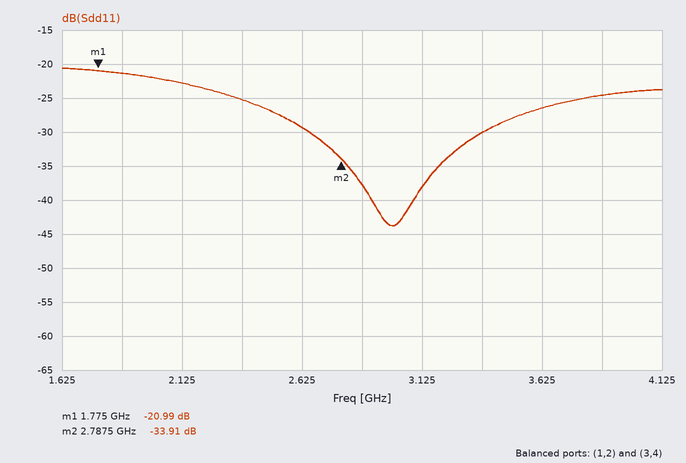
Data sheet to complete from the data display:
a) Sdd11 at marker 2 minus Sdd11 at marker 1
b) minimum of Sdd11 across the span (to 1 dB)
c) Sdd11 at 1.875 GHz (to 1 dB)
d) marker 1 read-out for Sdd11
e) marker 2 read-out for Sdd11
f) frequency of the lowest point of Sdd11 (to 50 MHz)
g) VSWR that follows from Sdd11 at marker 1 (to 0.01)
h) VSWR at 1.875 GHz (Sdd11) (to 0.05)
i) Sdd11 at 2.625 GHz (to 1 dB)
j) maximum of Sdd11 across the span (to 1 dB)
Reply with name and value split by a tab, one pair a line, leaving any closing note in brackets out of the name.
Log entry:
Sdd11 at marker 2 minus Sdd11 at marker 1	-12.92 dB
minimum of Sdd11 across the span	-44 dB
Sdd11 at 1.875 GHz	-21 dB
marker 1 read-out for Sdd11	-20.99 dB
marker 2 read-out for Sdd11	-33.91 dB
frequency of the lowest point of Sdd11	3.00 GHz
VSWR that follows from Sdd11 at marker 1	1.20
VSWR at 1.875 GHz (Sdd11)	1.20
Sdd11 at 2.625 GHz	-29 dB
maximum of Sdd11 across the span	-21 dB
